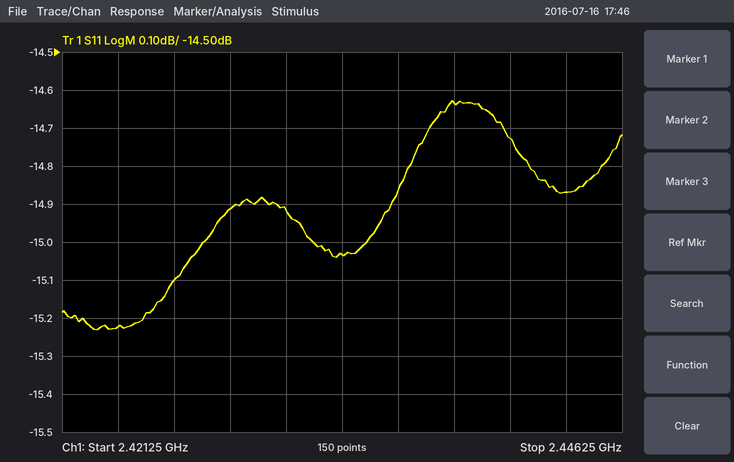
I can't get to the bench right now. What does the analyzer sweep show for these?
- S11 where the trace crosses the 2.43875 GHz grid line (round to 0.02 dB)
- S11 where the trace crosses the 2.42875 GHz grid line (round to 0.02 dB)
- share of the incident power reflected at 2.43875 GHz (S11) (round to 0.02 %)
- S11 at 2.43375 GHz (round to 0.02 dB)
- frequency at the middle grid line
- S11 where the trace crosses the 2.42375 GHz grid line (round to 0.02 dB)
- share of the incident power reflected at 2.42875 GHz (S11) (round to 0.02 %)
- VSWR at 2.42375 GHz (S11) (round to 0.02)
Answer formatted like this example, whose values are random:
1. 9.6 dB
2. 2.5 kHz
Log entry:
1. -14.64 dB
2. -14.92 dB
3. 3.44 %
4. -15.04 dB
5. 2.43375 GHz
6. -15.22 dB
7. 3.22 %
8. 1.42
